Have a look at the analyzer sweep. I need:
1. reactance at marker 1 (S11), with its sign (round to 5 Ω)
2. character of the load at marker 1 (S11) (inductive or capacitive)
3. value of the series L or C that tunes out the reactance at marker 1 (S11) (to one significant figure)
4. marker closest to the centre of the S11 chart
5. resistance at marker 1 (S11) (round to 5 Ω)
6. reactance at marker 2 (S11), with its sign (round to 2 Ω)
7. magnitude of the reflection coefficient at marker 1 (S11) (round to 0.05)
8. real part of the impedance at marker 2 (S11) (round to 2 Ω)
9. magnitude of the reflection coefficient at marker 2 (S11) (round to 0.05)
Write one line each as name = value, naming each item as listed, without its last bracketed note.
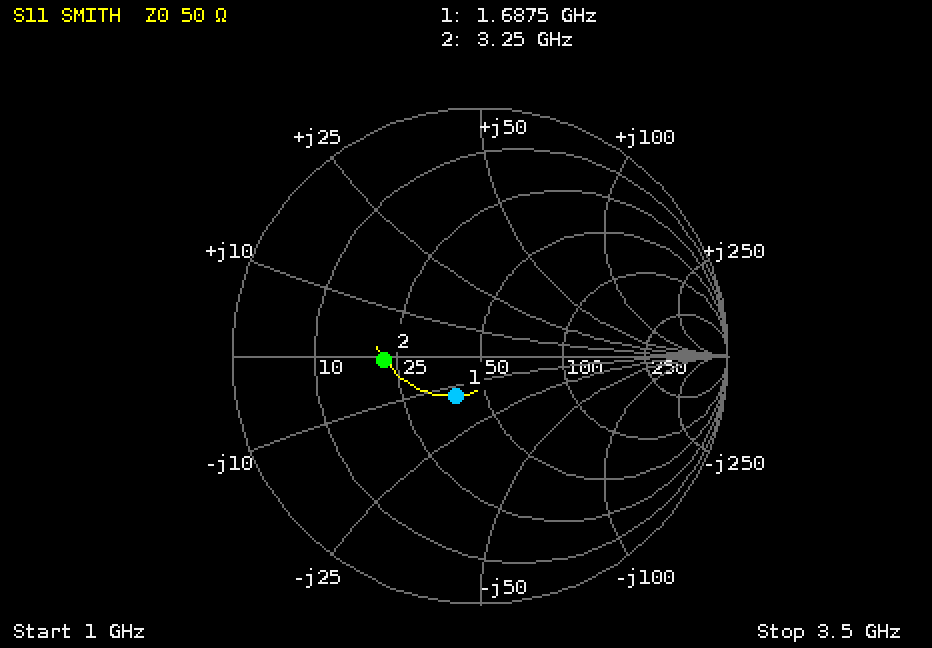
reactance at marker 1 (S11), with its sign = -15 Ω
character of the load at marker 1 (S11) = capacitive
value of the series L or C that tunes out the reactance at marker 1 (S11) = 1 nH
marker closest to the centre of the S11 chart = marker 1
resistance at marker 1 (S11) = 40 Ω
reactance at marker 2 (S11), with its sign = 0 Ω
magnitude of the reflection coefficient at marker 1 (S11) = 0.20
real part of the impedance at marker 2 (S11) = 22 Ω
magnitude of the reflection coefficient at marker 2 (S11) = 0.40
